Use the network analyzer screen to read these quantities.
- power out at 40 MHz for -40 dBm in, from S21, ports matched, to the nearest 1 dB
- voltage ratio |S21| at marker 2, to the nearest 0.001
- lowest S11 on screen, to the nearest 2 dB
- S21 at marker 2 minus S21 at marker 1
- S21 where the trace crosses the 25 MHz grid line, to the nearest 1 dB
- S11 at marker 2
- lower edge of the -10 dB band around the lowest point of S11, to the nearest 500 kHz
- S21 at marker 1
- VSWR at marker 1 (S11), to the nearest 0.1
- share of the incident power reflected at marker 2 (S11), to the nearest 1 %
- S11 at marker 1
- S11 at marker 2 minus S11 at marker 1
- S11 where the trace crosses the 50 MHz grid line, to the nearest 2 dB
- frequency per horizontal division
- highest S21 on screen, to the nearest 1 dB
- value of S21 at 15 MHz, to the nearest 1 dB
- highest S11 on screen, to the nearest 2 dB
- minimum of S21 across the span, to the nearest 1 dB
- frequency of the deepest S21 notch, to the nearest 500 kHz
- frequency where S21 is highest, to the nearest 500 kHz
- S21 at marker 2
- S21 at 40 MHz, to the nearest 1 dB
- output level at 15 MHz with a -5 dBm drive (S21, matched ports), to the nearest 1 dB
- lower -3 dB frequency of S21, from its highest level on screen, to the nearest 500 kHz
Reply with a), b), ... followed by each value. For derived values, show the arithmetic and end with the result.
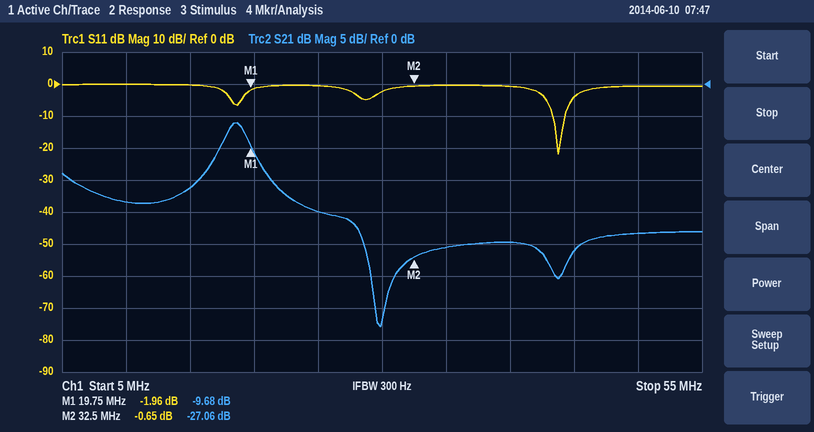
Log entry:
a) -40 dBm + (-25 dB) = -65 dBm
b) 10^(-27.06/20) ≈ 0.044
c) -22 dB
d) -27.06 − (-9.68) = -17.38 dB
e) -20 dB
f) -0.65 dB
g) 43.5 MHz
h) -9.68 dB
i) (1 + 0.7980)/(1 − 0.7980) ≈ 8.9
j) 10^(-0.65/10) ≈ 86 %
k) -1.96 dB
l) -0.65 − (-1.96) = 1.31 dB
m) 0 dB
n) 5 MHz
o) -6 dB
p) -16 dB
q) 0 dB
r) -38 dB
s) 30.0 MHz
t) 18.5 MHz
u) -27.06 dB
v) -25 dB
w) -5 dBm + (-16 dB) = -21 dBm
x) 17.5 MHz
